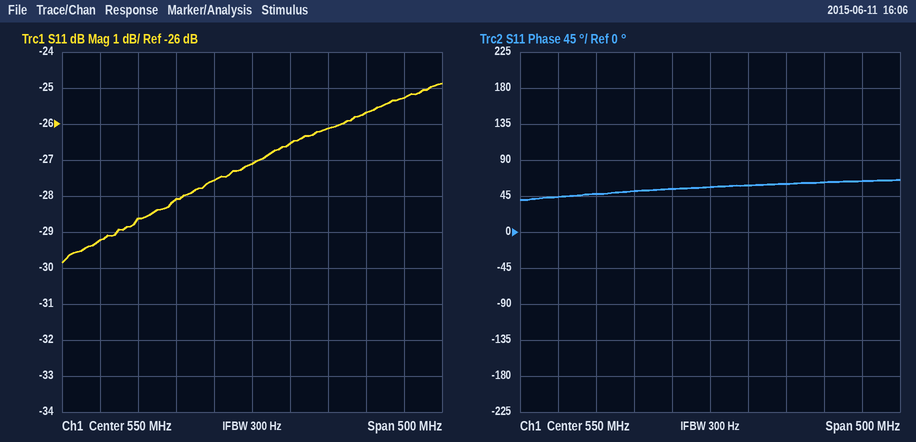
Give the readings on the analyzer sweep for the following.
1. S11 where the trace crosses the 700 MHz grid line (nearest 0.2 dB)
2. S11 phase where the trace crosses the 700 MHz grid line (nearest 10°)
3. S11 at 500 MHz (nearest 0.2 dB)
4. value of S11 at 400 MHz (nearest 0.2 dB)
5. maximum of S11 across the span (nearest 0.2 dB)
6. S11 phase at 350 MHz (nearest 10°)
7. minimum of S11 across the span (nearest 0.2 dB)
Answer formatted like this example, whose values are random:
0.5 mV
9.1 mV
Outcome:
-25.6 dB
60°
-27.6 dB
-28.6 dB
-24.8 dB
40°
-29.8 dB
